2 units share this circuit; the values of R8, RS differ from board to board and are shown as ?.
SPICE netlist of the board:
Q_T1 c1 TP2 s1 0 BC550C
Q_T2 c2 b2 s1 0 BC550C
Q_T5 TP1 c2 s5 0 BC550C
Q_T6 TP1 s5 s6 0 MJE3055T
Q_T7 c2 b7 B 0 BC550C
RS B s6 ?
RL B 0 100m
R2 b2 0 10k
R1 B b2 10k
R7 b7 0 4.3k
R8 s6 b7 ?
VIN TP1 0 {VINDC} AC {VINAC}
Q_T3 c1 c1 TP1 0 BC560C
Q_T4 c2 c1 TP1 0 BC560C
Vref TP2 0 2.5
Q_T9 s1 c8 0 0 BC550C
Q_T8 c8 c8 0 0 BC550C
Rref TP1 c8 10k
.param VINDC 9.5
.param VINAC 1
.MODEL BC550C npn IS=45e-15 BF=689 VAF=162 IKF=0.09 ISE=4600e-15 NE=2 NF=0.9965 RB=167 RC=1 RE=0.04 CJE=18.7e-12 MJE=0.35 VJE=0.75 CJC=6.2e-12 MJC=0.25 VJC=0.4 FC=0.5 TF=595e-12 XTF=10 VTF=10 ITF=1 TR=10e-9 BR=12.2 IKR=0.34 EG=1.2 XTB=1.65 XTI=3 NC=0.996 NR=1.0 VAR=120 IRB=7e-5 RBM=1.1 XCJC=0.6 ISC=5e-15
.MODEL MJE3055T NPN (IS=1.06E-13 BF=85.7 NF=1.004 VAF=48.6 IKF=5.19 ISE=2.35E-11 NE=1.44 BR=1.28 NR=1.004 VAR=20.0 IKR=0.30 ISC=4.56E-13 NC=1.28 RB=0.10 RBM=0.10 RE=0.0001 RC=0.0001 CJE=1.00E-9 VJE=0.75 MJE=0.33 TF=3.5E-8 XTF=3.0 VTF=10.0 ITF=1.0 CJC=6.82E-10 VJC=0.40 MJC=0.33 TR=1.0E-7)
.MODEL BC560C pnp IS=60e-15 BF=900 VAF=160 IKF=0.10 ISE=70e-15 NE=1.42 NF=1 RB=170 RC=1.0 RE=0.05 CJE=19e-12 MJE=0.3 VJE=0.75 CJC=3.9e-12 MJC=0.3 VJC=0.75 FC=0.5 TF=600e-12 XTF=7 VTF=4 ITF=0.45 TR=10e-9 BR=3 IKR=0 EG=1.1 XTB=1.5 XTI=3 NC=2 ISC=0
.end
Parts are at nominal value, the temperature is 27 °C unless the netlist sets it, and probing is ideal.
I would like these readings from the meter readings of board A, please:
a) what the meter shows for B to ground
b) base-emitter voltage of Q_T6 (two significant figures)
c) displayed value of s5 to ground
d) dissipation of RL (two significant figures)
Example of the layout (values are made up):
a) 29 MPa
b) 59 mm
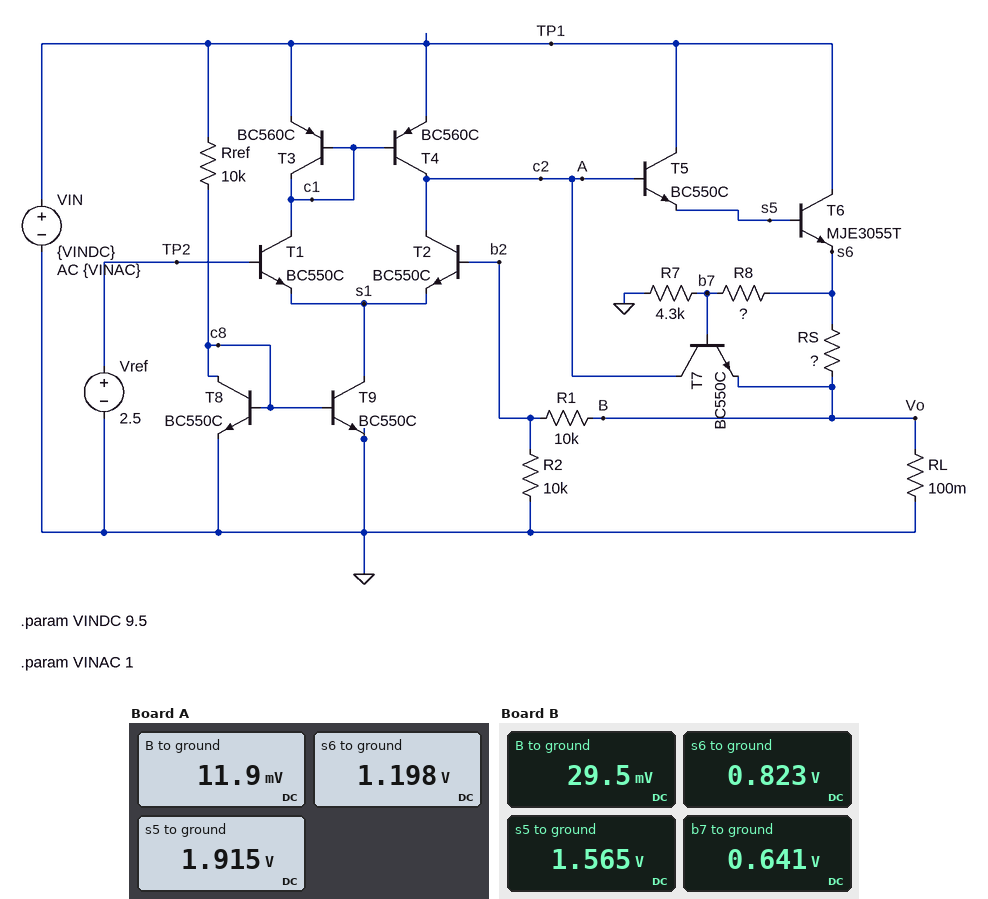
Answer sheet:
a) 11.9 mV
b) 720 mV
c) 1.915 V
d) 1.4 mW
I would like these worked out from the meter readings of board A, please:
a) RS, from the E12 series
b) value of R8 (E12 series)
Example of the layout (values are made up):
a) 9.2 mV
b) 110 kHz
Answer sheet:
a) 10 Ω
b) 3.9 kΩ
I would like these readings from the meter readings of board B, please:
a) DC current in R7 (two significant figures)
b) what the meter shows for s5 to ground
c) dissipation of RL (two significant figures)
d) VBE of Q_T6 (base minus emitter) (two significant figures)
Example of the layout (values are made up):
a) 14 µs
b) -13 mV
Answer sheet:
a) 150 µA
b) 1.565 V
c) 8.7 mW
d) 740 mV
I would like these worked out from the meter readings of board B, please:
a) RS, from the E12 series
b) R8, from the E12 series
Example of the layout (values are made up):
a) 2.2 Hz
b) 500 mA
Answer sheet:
a) 2.7 Ω
b) 1.2 kΩ
